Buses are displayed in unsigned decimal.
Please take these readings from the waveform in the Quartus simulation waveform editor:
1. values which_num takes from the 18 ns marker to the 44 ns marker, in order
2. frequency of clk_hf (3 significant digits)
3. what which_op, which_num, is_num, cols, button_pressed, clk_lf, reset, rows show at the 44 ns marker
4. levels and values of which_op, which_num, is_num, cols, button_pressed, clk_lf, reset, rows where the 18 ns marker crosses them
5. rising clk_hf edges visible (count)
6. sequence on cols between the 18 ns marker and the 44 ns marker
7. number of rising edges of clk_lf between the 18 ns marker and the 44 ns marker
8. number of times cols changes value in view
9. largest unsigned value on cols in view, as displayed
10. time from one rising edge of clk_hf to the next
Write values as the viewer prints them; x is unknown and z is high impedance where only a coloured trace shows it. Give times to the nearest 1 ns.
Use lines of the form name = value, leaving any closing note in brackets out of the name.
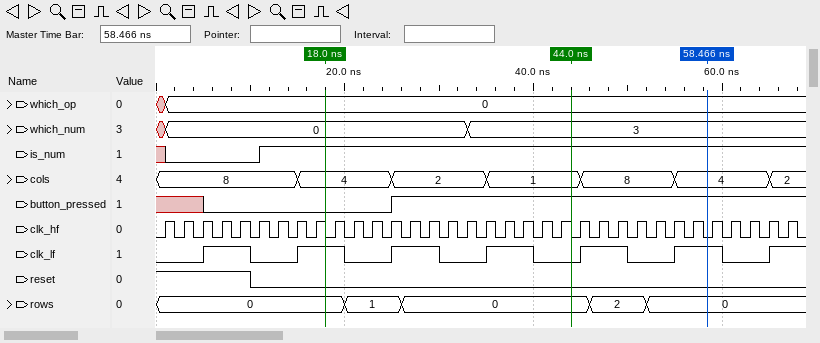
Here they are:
values which_num takes from the 18 ns marker to the 44 ns marker, in order = 0, 3
frequency of clk_hf = 500 MHz
what which_op, which_num, is_num, cols, button_pressed, clk_lf, reset, rows show at the 44 ns marker = which_op=0, which_num=3, is_num=1, cols=1, button_pressed=1, clk_lf=0, reset=0, rows=0
levels and values of which_op, which_num, is_num, cols, button_pressed, clk_lf, reset, rows where the 18 ns marker crosses them = which_op=0, which_num=0, is_num=1, cols=4, button_pressed=0, clk_lf=1, reset=0, rows=0
rising clk_hf edges visible = 34
sequence on cols between the 18 ns marker and the 44 ns marker = 4, 2, 1
number of rising edges of clk_lf between the 18 ns marker and the 44 ns marker = 2
number of times cols changes value in view = 6
largest unsigned value on cols in view, as displayed = 8
time from one rising edge of clk_hf to the next = 2 ns
